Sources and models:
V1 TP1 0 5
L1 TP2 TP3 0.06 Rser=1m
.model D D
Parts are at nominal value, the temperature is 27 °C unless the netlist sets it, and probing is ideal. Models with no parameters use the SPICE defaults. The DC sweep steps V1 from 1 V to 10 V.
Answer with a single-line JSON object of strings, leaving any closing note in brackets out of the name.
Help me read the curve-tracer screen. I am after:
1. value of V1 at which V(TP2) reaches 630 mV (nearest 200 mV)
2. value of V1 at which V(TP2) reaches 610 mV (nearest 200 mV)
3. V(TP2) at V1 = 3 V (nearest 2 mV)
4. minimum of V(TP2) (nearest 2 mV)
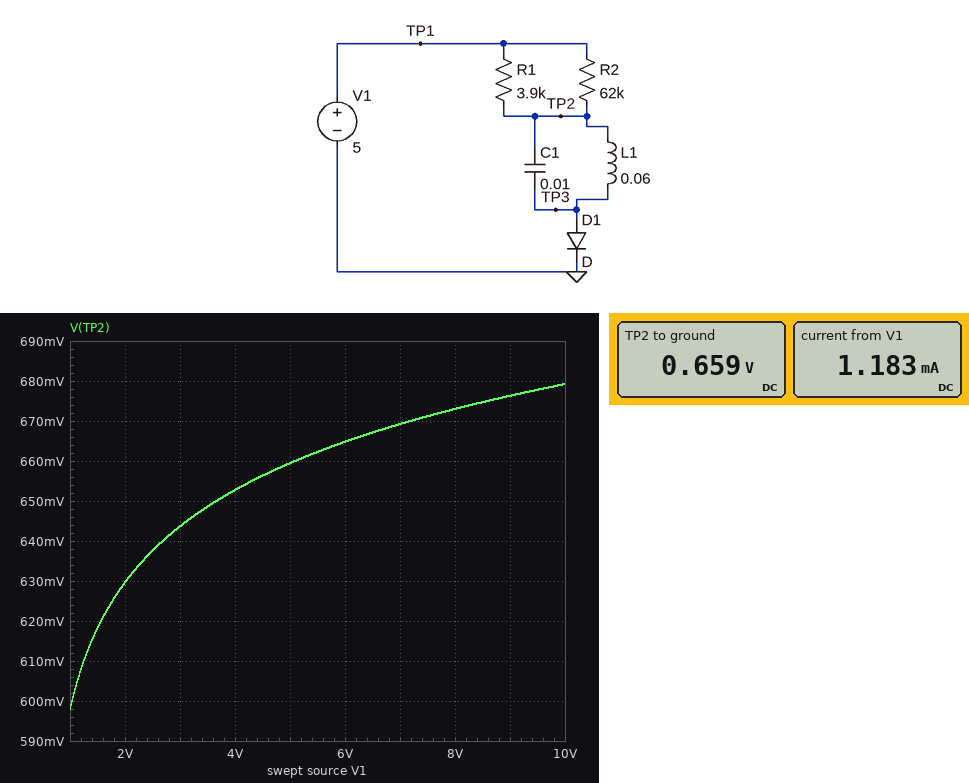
{"value of V1 at which V(TP2) reaches 630 mV": "2.0 V", "value of V1 at which V(TP2) reaches 610 mV": "1.2 V", "V(TP2) at V1 = 3 V": "644 mV", "minimum of V(TP2)": "598 mV"}
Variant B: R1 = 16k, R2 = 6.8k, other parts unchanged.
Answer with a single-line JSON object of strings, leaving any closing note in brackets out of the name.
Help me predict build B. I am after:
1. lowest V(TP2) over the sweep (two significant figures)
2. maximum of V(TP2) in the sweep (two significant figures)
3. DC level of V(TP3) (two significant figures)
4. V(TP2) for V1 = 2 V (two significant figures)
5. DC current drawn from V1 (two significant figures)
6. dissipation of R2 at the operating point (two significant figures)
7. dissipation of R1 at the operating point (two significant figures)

{"lowest V(TP2) over the sweep": "590 mV", "maximum of V(TP2) in the sweep": "670 mV", "DC level of V(TP3)": "650 mV", "V(TP2) for V1 = 2 V": "620 mV", "DC current drawn from V1": "910 µA", "dissipation of R2 at the operating point": "2.8 mW", "dissipation of R1 at the operating point": "1.2 mW"}
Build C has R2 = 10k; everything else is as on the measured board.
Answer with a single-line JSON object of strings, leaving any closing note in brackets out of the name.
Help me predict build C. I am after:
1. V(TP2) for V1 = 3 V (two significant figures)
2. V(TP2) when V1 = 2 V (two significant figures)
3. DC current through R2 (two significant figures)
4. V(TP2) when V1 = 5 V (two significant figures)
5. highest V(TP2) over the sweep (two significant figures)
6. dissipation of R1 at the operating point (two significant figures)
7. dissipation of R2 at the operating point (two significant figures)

{"V(TP2) for V1 = 3 V": "650 mV", "V(TP2) when V1 = 2 V": "640 mV", "DC current through R2": "430 µA", "V(TP2) when V1 = 5 V": "670 mV", "highest V(TP2) over the sweep": "690 mV", "dissipation of R1 at the operating point": "4.8 mW", "dissipation of R2 at the operating point": "1.9 mW"}
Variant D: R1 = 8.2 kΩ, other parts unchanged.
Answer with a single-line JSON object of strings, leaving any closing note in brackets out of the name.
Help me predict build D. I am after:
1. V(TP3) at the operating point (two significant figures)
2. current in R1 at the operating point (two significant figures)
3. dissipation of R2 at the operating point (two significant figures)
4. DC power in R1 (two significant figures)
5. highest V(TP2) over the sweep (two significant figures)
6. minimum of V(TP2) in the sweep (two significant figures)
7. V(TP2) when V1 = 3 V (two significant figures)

{"V(TP3) at the operating point": "640 mV", "current in R1 at the operating point": "530 µA", "dissipation of R2 at the operating point": "310 µW", "DC power in R1": "2.3 mW", "highest V(TP2) over the sweep": "660 mV", "minimum of V(TP2) in the sweep": "580 mV", "V(TP2) when V1 = 3 V": "630 mV"}
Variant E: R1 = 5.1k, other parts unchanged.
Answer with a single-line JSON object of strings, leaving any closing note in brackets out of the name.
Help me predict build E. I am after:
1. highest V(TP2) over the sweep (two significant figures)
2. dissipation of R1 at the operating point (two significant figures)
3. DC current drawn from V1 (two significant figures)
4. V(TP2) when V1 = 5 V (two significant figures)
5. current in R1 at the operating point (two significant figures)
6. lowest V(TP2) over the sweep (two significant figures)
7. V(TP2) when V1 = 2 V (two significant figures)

{"highest V(TP2) over the sweep": "670 mV", "dissipation of R1 at the operating point": "3.7 mW", "DC current drawn from V1": "920 µA", "V(TP2) when V1 = 5 V": "650 mV", "current in R1 at the operating point": "850 µA", "lowest V(TP2) over the sweep": "590 mV", "V(TP2) when V1 = 2 V": "620 mV"}
